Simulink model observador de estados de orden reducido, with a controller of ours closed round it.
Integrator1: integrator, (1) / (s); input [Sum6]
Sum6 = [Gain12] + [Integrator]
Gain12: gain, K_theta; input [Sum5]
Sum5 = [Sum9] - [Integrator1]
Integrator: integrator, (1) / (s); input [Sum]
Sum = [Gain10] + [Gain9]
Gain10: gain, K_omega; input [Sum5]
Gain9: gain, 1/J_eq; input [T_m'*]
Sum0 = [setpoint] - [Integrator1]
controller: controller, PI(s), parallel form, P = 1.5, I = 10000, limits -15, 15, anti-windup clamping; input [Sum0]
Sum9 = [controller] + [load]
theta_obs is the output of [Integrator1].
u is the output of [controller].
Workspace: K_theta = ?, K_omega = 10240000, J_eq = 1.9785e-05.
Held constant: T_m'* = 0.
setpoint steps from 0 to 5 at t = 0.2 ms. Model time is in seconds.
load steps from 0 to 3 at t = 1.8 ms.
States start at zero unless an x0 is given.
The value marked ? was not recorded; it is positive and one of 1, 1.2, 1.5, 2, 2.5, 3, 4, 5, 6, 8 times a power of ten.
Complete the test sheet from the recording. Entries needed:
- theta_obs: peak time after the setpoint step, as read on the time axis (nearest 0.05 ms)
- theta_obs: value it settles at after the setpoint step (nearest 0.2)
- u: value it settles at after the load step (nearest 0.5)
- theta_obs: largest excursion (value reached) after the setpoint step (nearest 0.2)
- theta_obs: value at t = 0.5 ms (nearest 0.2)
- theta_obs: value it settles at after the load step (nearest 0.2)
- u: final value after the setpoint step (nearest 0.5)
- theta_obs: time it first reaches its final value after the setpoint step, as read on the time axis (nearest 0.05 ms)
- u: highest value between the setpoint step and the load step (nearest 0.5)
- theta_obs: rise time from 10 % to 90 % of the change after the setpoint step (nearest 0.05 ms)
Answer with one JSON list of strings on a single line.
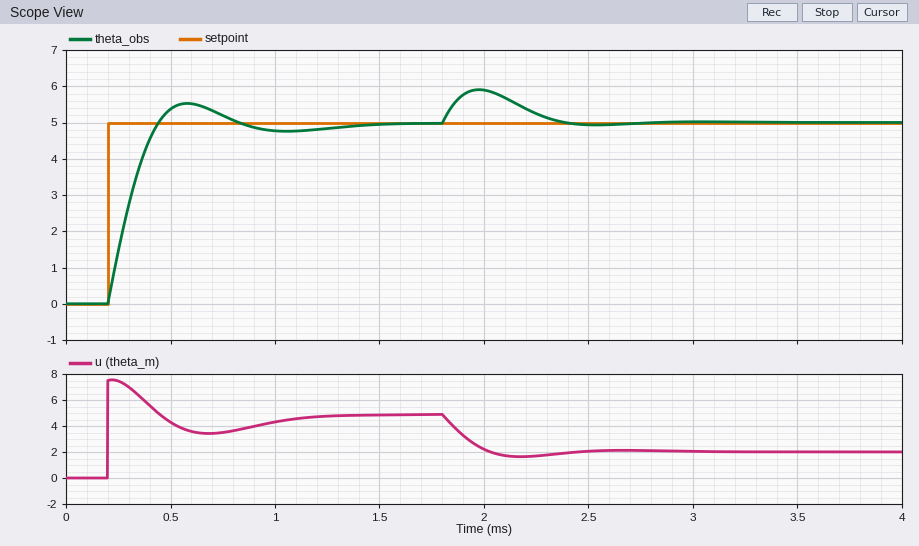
["0.60 ms", "5.0", "2.0", "5.6", "5.4", "5.0", "5.0", "0.45 ms", "7.5", "0.20 ms"]
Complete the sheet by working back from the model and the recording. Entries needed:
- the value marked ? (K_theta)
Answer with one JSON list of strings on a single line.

["4000"]
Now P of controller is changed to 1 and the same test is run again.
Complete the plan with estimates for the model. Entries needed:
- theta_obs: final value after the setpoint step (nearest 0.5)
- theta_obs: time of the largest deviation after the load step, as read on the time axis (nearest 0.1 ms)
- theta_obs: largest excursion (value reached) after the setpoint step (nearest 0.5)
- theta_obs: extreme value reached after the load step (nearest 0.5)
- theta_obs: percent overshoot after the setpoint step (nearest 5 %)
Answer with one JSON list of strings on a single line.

["5.0", "2.0 ms", "6.0", "6.0", "20 %"]
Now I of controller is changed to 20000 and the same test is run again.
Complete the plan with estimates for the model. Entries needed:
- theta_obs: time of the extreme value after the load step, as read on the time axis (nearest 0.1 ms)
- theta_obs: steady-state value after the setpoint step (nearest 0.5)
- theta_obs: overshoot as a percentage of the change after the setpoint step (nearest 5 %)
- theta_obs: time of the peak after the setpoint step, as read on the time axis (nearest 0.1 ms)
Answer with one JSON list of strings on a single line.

["1.9 ms", "5.0", "25 %", "0.5 ms"]
